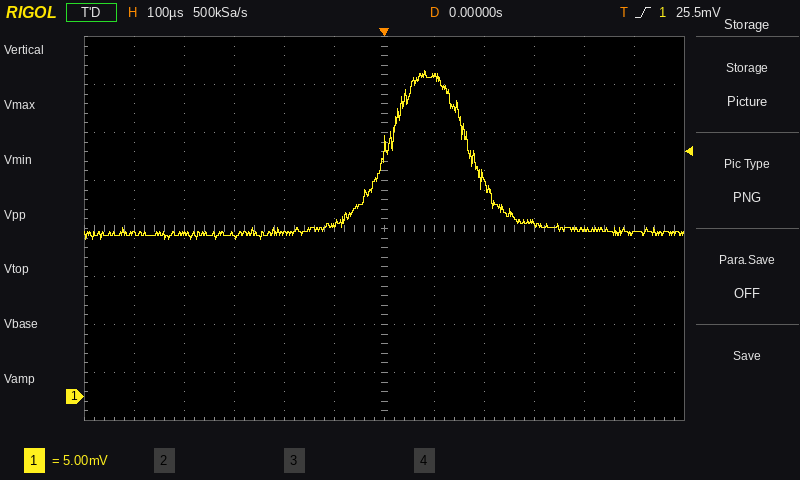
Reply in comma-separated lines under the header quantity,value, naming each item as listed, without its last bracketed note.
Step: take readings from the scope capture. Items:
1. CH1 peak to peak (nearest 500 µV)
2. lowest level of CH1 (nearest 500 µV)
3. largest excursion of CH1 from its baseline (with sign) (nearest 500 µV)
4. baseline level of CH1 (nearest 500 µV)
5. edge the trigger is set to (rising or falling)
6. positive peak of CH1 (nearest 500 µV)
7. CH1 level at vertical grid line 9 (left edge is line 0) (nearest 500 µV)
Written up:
quantity,value
CH1 peak to peak,17.5 mV
lowest level of CH1,16.5 mV
largest excursion of CH1 from its baseline (with sign),+17.0 mV
baseline level of CH1,17.0 mV
edge the trigger is set to,rising
positive peak of CH1,34.0 mV
CH1 level at vertical grid line 9 (left edge is line 0),18.0 mV
